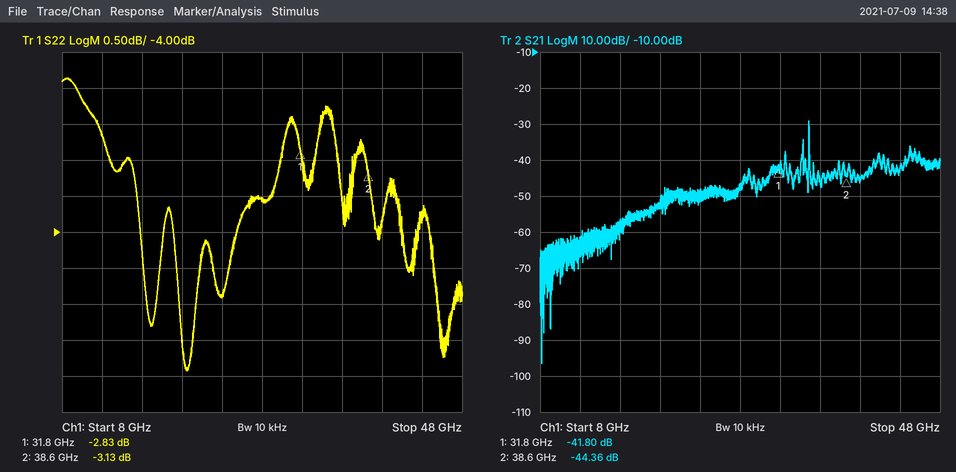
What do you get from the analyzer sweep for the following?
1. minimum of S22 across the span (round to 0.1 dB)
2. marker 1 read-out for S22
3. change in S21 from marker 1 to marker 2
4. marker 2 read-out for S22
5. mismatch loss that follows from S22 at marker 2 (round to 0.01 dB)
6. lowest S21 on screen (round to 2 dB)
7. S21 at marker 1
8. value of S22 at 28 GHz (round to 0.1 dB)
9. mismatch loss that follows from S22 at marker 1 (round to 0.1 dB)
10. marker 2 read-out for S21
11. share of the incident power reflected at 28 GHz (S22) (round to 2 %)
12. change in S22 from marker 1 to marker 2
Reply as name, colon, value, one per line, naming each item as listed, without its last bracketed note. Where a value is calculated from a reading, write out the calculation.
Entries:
minimum of S22 across the span: -5.9 dB
marker 1 read-out for S22: -2.83 dB
change in S21 from marker 1 to marker 2: -44.36 − (-41.8) = -2.56 dB
marker 2 read-out for S22: -3.13 dB
mismatch loss that follows from S22 at marker 2: −10 log10(1 − 10^(-3.13/10)) ≈ 2.89 dB
lowest S21 on screen: -96 dB
S21 at marker 1: -41.80 dB
value of S22 at 28 GHz: -3.5 dB
mismatch loss that follows from S22 at marker 1: −10 log10(1 − 10^(-2.83/10)) ≈ 3.2 dB
marker 2 read-out for S21: -44.36 dB
share of the incident power reflected at 28 GHz (S22): 10^(-3.5/10) ≈ 44.7 %, so 44 % to the nearest 2 %
change in S22 from marker 1 to marker 2: -3.13 − (-2.83) = -0.30 dB
